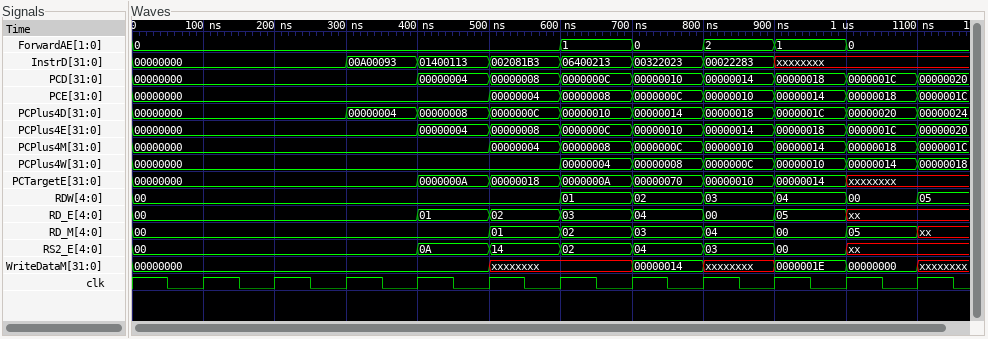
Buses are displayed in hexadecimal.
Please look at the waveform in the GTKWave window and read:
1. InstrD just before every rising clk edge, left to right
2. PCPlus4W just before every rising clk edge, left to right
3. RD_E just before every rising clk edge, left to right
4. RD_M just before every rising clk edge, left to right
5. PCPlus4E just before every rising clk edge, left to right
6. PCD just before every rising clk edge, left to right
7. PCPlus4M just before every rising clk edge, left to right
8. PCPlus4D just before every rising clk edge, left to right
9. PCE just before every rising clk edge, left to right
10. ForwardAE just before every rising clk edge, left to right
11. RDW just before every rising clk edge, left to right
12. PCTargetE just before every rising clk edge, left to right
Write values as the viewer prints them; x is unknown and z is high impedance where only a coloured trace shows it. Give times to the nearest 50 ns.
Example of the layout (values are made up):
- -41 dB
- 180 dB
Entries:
- 00000000, 00000000, 00000000, 00A00093, 01400113, 002081B3, 06400213, 00322023, 00022283, xxxxxxxx, xxxxxxxx
- 00000000, 00000000, 00000000, 00000000, 00000000, 00000000, 00000004, 00000008, 0000000C, 00000010, 00000014
- 00, 00, 00, 00, 01, 02, 03, 04, 00, 05, xx
- 00, 00, 00, 00, 00, 01, 02, 03, 04, 00, 05
- 00000000, 00000000, 00000000, 00000000, 00000004, 00000008, 0000000C, 00000010, 00000014, 00000018, 0000001C
- 00000000, 00000000, 00000000, 00000000, 00000004, 00000008, 0000000C, 00000010, 00000014, 00000018, 0000001C
- 00000000, 00000000, 00000000, 00000000, 00000000, 00000004, 00000008, 0000000C, 00000010, 00000014, 00000018
- 00000000, 00000000, 00000000, 00000004, 00000008, 0000000C, 00000010, 00000014, 00000018, 0000001C, 00000020
- 00000000, 00000000, 00000000, 00000000, 00000000, 00000004, 00000008, 0000000C, 00000010, 00000014, 00000018
- 0, 0, 0, 0, 0, 0, 1, 0, 2, 1, 0
- 00, 00, 00, 00, 00, 00, 01, 02, 03, 04, 00
- 00000000, 00000000, 00000000, 00000000, 0000000A, 00000018, 0000000A, 00000070, 00000010, 00000014, xxxxxxxx
